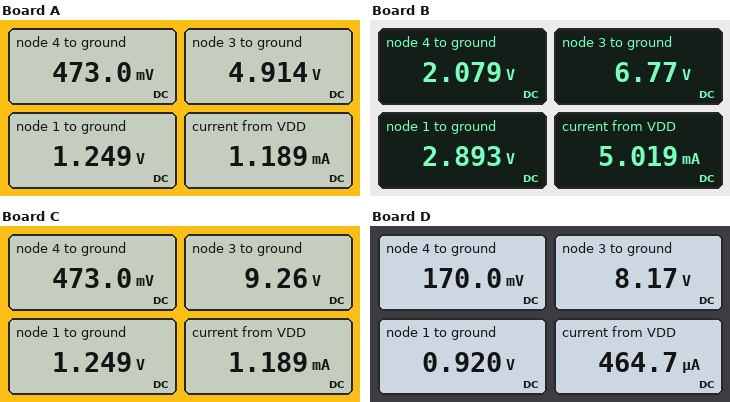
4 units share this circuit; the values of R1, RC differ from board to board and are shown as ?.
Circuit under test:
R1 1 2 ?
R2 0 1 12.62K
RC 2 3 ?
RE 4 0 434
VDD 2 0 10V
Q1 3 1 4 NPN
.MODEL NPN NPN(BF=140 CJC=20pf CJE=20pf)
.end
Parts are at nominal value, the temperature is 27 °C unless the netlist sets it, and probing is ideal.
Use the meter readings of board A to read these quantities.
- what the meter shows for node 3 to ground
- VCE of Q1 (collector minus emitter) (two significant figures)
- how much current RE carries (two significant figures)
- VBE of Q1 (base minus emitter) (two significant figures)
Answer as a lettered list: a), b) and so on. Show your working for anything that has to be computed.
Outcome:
a) 4.914 V
b) 4.914 V - 473 mV = 4.4 V
c) (473 mV) / 434 Ω = 1.1 mA
d) 1.249 V - 473 mV = 780 mV
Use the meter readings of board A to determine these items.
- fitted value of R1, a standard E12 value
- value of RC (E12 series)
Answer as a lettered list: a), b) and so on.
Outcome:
a) 82 kΩ
b) 4.7 kΩ
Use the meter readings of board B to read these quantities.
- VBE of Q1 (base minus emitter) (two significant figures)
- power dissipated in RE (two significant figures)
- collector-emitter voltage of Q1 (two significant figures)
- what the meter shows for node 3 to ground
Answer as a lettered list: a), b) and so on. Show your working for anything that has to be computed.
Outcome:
a) 2.893 V - 2.079 V = 810 mV
b) (2.079 V)^2 / 434 Ω = 10 mW
c) 6.77 V - 2.079 V = 4.7 V
d) 6.77 V
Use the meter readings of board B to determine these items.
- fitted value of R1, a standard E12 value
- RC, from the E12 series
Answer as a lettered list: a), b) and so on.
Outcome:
a) 27 kΩ
b) 680 Ω
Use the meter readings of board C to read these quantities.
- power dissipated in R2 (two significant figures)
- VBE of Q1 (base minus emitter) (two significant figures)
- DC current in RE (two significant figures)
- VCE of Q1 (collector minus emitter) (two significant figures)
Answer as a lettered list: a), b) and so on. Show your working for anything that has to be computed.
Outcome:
a) (1.249 V)^2 / 12.62 kΩ = 120 µW
b) 1.249 V - 473 mV = 780 mV
c) (473 mV) / 434 Ω = 1.1 mA
d) 9.26 V - 473 mV = 8.8 V
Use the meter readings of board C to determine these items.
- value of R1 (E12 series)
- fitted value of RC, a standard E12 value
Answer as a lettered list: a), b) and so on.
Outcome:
a) 82 kΩ
b) 680 Ω
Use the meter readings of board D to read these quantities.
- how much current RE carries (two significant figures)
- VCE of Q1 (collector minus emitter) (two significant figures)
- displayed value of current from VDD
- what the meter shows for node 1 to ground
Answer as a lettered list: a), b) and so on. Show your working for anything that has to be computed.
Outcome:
a) (170 mV) / 434 Ω = 390 µA
b) 8.17 V - 170 mV = 8.0 V
c) 464.7 µA
d) 0.920 V
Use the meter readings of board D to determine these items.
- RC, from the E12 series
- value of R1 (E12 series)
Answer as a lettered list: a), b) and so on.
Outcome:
a) 4.7 kΩ
b) 120 kΩ
